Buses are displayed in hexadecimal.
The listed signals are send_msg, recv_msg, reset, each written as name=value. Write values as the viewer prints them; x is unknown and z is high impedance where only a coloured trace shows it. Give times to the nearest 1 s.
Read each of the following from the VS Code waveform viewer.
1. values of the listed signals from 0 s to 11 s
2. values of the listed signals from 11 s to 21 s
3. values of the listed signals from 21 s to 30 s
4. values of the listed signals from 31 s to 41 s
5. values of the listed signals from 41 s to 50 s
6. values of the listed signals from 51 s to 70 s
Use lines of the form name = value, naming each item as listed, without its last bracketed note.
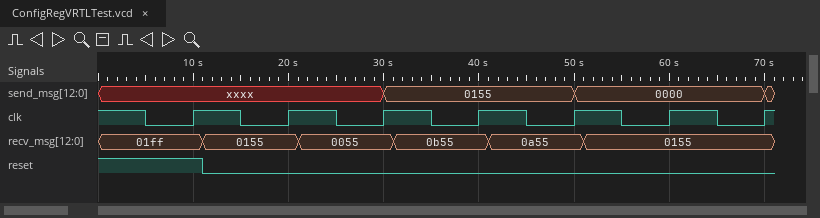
values of the listed signals from 0 s to 11 s = send_msg=xxxx, recv_msg=01ff, reset=1
values of the listed signals from 11 s to 21 s = send_msg=xxxx, recv_msg=0155, reset=0
values of the listed signals from 21 s to 30 s = send_msg=xxxx, recv_msg=0055, reset=0
values of the listed signals from 31 s to 41 s = send_msg=0155, recv_msg=0b55, reset=0
values of the listed signals from 41 s to 50 s = send_msg=0155, recv_msg=0a55, reset=0
values of the listed signals from 51 s to 70 s = send_msg=0000, recv_msg=0155, reset=0
